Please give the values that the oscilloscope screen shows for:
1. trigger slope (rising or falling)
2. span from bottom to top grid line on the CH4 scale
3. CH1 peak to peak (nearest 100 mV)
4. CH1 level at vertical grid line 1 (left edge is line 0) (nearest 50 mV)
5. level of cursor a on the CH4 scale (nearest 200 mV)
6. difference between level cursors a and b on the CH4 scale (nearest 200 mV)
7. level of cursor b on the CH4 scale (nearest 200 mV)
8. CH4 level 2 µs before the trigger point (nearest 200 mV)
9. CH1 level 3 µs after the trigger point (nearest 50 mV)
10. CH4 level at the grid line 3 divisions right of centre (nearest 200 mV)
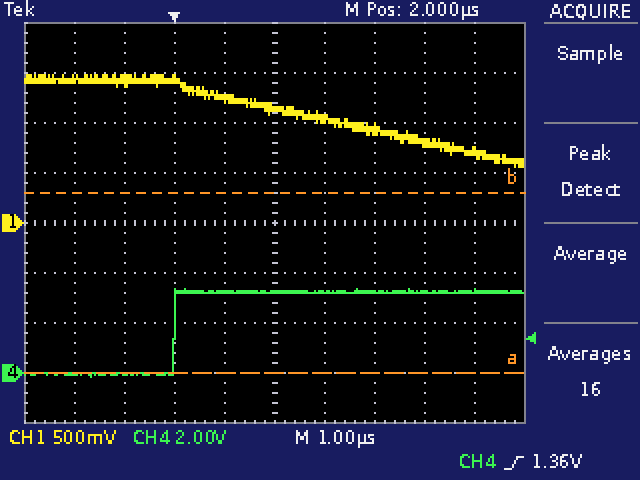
rising
16 V
900 mV
1.45 V
0.0 V
7.2 V
7.2 V
0.0 V
1.05 V
3.2 V
